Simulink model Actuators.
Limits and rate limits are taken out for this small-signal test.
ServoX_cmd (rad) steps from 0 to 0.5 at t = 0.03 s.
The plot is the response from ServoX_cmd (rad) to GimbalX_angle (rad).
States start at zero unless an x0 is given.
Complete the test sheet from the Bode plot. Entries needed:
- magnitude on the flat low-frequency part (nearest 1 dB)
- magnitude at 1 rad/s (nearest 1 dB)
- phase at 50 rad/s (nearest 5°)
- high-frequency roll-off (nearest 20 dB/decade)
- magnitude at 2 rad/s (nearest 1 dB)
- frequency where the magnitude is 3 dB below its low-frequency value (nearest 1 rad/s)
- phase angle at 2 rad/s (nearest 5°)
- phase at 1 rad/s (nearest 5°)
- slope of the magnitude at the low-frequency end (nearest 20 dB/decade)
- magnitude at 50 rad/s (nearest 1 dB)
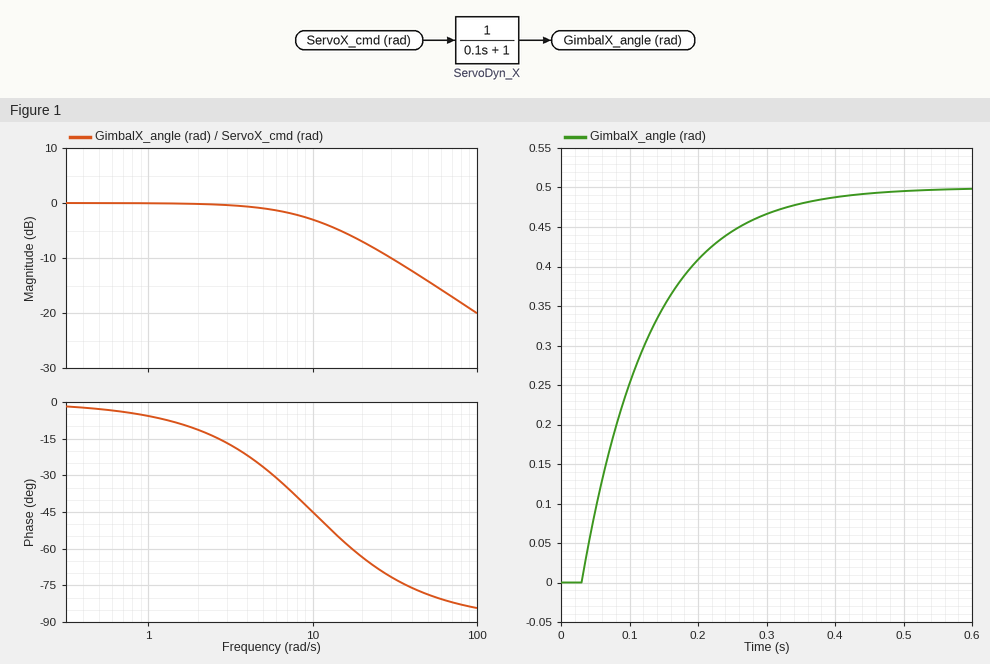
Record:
0 dB
0 dB
-80°
-20 dB/decade
0 dB
10 rad/s
-10°
-5°
0 dB/decade
-14 dB
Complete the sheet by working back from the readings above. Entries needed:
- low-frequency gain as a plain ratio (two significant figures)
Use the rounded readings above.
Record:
1.0
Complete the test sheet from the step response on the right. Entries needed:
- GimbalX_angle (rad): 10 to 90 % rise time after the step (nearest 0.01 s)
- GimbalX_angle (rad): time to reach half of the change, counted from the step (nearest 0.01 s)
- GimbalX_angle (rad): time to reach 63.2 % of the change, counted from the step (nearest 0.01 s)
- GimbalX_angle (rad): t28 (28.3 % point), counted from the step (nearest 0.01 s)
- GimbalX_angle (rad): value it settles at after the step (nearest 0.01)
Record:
0.22 s
0.07 s
0.10 s
0.03 s
0.50
